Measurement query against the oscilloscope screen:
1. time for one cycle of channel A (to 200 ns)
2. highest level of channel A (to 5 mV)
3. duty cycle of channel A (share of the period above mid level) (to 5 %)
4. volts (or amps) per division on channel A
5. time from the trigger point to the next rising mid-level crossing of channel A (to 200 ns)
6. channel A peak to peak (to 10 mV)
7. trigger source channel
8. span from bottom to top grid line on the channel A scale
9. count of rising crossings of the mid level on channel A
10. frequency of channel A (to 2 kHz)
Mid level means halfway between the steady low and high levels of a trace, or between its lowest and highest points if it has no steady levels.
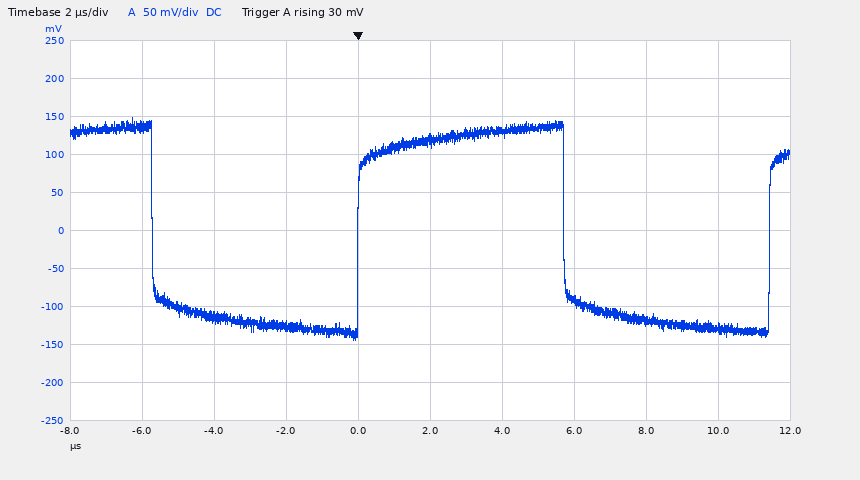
11.4 µs
150 mV
50 %
50 mV
11.4 µs
290 mV
channel A
500 mV
2
88 kHz
